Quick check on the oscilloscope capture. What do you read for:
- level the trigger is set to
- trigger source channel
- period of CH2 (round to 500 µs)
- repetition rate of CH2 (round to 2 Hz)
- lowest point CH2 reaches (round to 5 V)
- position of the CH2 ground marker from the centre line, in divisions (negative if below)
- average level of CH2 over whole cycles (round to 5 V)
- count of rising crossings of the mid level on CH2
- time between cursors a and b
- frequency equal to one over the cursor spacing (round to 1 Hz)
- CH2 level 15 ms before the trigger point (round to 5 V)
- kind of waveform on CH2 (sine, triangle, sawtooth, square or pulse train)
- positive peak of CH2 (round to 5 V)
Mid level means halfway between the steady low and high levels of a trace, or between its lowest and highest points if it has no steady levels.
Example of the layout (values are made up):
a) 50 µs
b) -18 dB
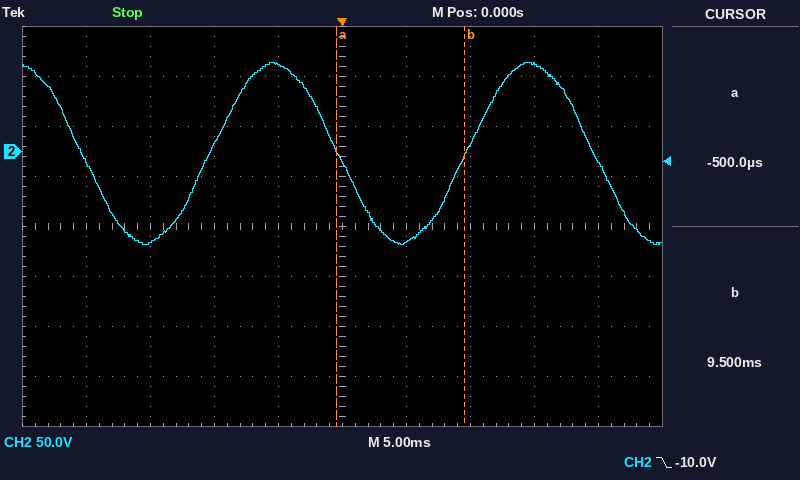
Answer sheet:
a) -10.0 V
b) CH2
c) 20.0 ms
d) 50 Hz
e) -95 V
f) +1.5 div
g) 0 V
h) 2
i) 10.0 ms
j) 100 Hz
k) -90 V
l) sine
m) 90 V
